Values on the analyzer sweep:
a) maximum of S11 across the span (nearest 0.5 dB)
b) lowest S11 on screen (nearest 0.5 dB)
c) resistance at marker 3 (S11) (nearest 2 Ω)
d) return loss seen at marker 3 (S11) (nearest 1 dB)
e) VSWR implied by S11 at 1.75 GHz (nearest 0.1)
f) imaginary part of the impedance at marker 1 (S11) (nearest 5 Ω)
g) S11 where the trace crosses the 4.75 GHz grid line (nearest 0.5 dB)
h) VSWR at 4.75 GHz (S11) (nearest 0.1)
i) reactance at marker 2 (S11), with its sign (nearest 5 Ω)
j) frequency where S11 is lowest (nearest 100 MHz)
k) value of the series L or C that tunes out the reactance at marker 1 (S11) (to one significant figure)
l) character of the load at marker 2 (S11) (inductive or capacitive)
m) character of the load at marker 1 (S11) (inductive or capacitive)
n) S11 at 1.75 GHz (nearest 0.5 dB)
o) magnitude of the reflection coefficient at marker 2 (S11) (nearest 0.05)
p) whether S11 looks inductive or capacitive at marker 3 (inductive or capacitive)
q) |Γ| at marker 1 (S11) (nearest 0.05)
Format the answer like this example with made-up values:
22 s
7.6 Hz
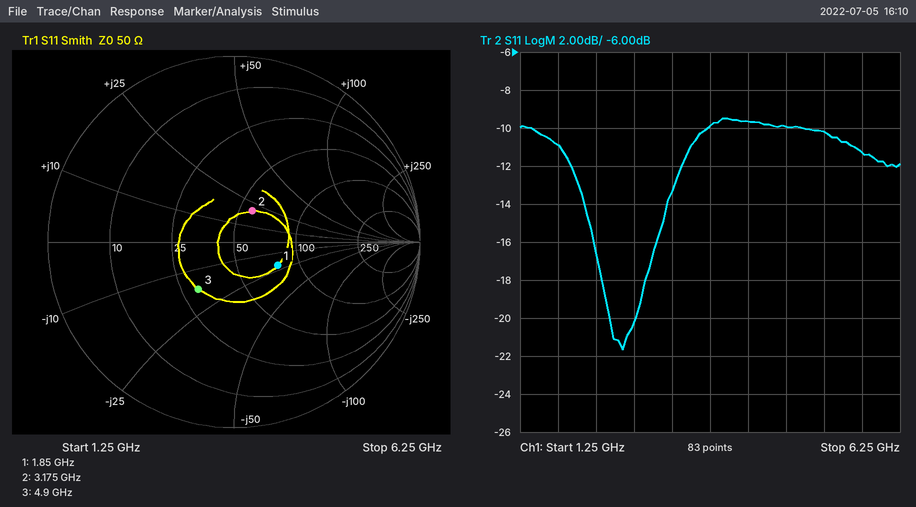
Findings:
-9.5 dB
-21.5 dB
30 Ω
10 dB
1.8
-20 Ω
-10.0 dB
1.9
+20 Ω
2.6 GHz
2 nH
inductive
capacitive
-11.0 dB
0.20
capacitive
0.25
